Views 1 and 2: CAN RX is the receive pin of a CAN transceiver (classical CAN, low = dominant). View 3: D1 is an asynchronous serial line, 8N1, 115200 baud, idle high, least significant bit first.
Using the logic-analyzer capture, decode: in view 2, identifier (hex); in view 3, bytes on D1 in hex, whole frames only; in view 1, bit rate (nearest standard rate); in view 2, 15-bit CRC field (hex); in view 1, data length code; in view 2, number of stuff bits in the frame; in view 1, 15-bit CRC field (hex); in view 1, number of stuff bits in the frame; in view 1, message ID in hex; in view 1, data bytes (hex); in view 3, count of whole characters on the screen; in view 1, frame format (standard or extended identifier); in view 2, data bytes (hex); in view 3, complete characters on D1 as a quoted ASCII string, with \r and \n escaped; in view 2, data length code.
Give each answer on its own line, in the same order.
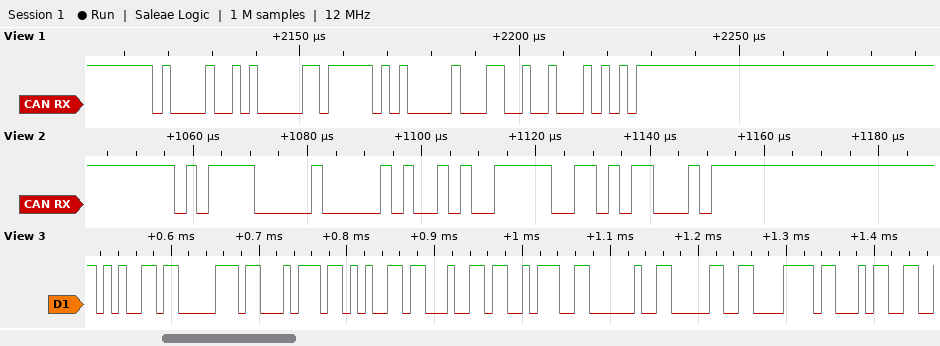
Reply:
0x5E0
65 70 74 65 64 3A 20 30 78 34
500 kbit/s
0x7B58
2
3
0x648A
3
0x425
FD 00
10
standard
29
"epted: 0x4"
1
